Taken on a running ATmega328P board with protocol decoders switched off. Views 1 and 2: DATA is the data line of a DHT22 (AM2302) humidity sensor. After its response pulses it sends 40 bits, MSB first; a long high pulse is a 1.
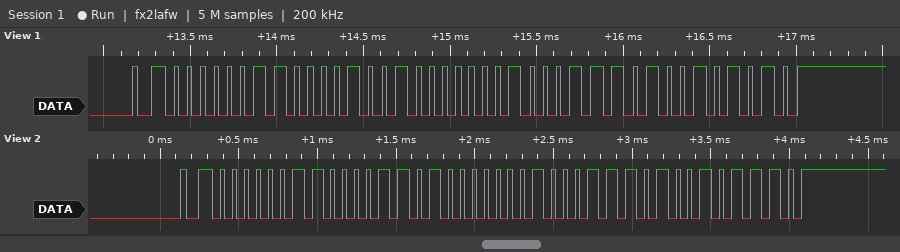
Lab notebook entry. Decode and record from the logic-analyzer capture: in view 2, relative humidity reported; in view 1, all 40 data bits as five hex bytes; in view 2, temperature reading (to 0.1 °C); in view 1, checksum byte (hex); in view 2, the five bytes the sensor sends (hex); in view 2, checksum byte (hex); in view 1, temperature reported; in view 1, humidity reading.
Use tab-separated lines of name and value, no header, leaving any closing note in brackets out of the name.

in view 2, relative humidity reported	78.1 %
in view 1, all 40 data bits as five hex bytes	03 09 01 1D 2A
in view 2, temperature reading	28.5 °C
in view 1, checksum byte	0x2A
in view 2, the five bytes the sensor sends	03 0D 01 1D 2E
in view 2, checksum byte	0x2E
in view 1, temperature reported	28.5 °C
in view 1, humidity reading	77.7 %
